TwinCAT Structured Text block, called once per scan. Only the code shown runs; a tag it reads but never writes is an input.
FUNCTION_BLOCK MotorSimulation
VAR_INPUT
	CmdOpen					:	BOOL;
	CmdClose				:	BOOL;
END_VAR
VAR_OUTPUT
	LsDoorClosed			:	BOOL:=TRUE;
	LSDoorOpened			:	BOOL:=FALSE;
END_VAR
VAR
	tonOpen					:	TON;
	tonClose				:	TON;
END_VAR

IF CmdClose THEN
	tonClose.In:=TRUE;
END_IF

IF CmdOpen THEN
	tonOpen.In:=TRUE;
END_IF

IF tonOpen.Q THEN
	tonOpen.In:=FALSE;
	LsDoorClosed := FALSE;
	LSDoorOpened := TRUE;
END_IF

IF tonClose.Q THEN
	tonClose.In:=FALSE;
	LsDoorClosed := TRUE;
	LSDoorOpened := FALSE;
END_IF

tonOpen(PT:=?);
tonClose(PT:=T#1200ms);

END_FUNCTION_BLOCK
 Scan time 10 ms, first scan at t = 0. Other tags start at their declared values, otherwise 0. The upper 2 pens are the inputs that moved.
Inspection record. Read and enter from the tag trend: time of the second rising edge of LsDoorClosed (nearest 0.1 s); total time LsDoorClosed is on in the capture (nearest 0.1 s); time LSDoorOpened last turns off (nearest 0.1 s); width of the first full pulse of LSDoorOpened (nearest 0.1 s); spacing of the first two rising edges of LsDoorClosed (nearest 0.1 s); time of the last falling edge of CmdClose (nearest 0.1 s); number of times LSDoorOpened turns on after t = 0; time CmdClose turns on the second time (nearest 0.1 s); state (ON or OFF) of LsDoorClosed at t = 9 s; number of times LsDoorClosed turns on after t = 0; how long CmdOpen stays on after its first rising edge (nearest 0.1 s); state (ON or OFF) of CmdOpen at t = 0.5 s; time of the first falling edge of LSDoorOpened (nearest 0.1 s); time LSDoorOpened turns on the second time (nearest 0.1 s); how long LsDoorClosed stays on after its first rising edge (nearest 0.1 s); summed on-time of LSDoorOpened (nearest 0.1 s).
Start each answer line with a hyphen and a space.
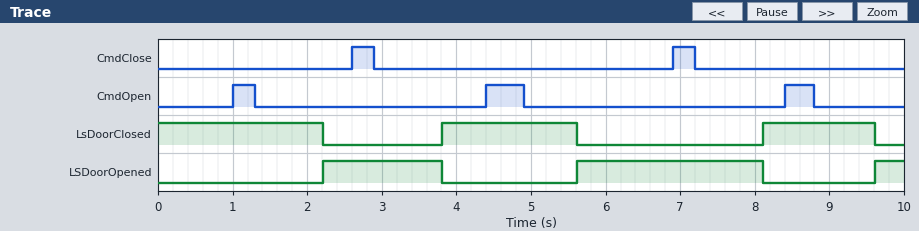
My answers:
- 8.1 s
- 5.5 s
- 8.1 s
- 1.6 s
- 4.3 s
- 7.2 s
- 3
- 6.9 s
- ON
- 2
- 0.3 s
- OFF
- 3.8 s
- 5.6 s
- 1.8 s
- 4.5 s
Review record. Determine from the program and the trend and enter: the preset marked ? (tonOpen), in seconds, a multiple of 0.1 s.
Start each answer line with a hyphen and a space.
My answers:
- 1.2 s
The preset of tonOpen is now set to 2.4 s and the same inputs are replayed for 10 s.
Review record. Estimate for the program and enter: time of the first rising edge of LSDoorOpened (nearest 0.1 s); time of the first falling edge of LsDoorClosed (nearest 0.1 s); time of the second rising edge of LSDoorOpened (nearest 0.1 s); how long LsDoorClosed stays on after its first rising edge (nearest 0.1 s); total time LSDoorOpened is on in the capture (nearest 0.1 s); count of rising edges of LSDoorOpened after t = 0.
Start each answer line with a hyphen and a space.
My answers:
- 3.4 s
- 3.4 s
- 6.8 s
- 3.0 s
- 1.7 s
- 2
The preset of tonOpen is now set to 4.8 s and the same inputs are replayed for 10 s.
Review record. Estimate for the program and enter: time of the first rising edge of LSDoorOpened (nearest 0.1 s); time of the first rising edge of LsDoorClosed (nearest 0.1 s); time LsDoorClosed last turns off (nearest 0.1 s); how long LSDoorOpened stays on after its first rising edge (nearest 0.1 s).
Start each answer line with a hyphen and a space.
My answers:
- 5.8 s
- 8.1 s
- 5.8 s
- 2.3 s
